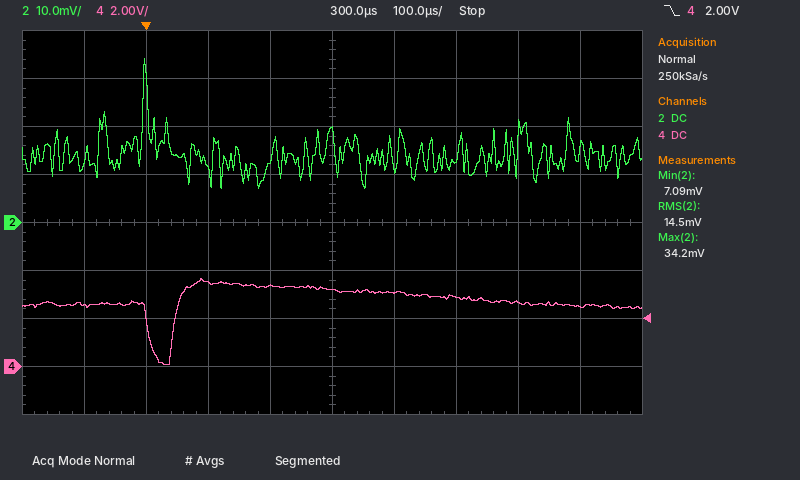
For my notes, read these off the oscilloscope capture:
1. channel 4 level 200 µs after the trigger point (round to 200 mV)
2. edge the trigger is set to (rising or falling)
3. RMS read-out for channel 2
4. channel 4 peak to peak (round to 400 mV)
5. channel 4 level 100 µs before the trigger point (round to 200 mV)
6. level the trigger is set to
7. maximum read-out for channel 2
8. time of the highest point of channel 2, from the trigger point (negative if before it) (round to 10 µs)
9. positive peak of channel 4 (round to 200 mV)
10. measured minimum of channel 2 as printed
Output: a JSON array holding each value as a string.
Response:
["3.4 V", "falling", "14.5 mV", "3.6 V", "2.6 V", "2.00 V", "34.2 mV", "0 µs", "3.6 V", "7.09 mV"]
